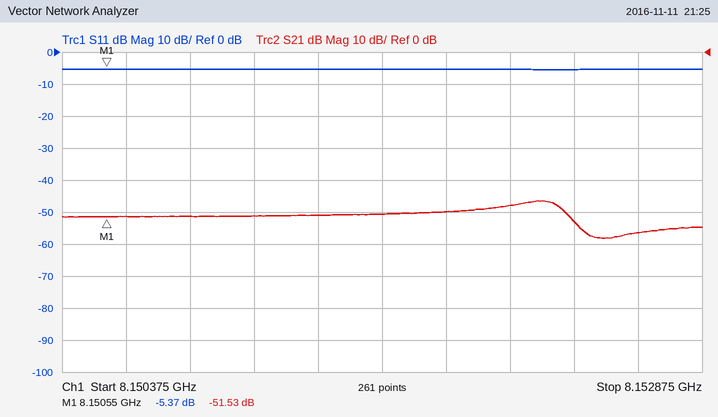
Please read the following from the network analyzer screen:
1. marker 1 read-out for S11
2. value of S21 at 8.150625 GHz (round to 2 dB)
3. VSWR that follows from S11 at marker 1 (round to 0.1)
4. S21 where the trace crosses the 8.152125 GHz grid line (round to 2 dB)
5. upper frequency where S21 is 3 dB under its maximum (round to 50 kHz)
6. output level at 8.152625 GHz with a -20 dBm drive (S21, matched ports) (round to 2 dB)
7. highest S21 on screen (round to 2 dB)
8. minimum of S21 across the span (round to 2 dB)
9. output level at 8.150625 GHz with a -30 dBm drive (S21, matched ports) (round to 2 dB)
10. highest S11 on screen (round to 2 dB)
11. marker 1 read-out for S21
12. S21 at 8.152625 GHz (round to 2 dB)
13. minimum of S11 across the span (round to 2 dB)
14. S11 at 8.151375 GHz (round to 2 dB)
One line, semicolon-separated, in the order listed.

-5.37 dB; -52 dB; 3.3; -48 dB; 8.15235 GHz; -76 dBm; -46 dB; -58 dB; -82 dBm; -6 dB; -51.53 dB; -56 dB; -6 dB; -6 dB
